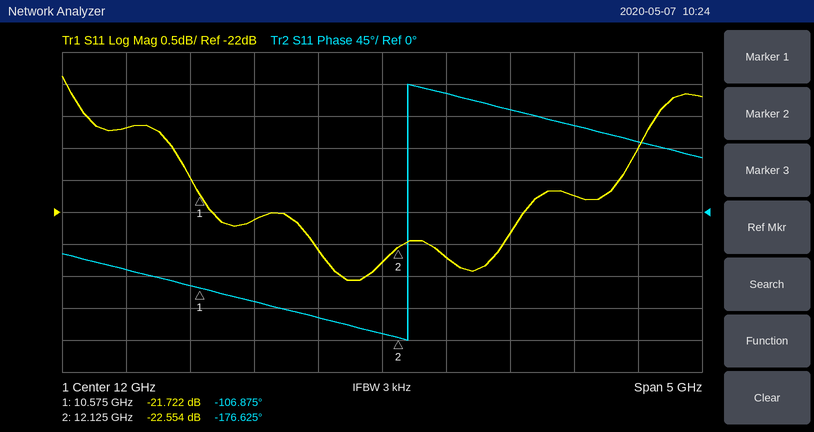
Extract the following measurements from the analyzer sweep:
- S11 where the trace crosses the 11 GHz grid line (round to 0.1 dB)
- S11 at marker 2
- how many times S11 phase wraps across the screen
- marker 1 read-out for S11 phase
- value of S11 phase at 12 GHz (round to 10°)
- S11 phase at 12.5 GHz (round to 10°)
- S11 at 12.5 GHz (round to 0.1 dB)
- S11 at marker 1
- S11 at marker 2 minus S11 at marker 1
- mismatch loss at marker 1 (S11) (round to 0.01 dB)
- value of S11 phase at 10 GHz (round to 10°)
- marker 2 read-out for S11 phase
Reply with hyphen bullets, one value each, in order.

- -22.1 dB
- -22.554 dB
- 1
- -106.875°
- -170°
- 170°
- -22.7 dB
- -21.722 dB
- -0.832 dB
- 0.03 dB
- -80°
- -176.625°
